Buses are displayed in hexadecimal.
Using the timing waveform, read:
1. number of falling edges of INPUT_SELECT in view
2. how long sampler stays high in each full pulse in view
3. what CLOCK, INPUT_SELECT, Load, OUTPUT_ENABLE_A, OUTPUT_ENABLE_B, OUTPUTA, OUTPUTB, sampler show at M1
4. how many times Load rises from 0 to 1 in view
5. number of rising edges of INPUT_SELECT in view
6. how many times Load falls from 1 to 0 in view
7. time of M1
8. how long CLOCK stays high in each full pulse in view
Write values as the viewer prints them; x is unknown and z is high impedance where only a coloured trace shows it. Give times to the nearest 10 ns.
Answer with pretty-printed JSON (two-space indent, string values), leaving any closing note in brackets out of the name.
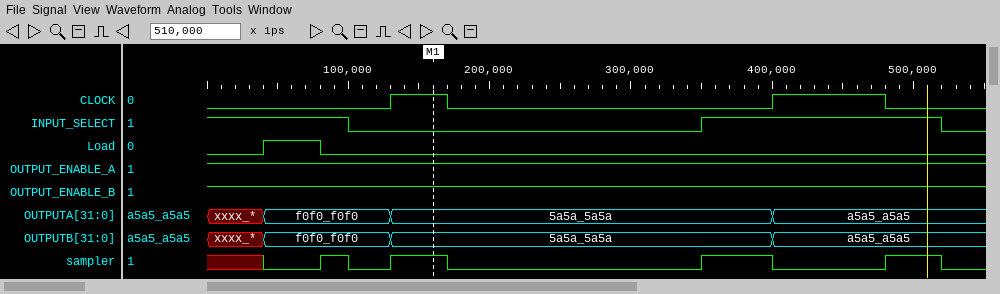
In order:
{
  "number of falling edges of INPUT_SELECT in view": "2",
  "how long sampler stays high in each full pulse in view": "20 ns, 40 ns, 50 ns, 40 ns",
  "what CLOCK, INPUT_SELECT, Load, OUTPUT_ENABLE_A, OUTPUT_ENABLE_B, OUTPUTA, OUTPUTB, sampler show at M1": "CLOCK=1, INPUT_SELECT=0, Load=0, OUTPUT_ENABLE_A=1, OUTPUT_ENABLE_B=1, OUTPUTA=5a5a_5a5a, OUTPUTB=5a5a_5a5a, sampler=1",
  "how many times Load rises from 0 to 1 in view": "1",
  "number of rising edges of INPUT_SELECT in view": "1",
  "how many times Load falls from 1 to 0 in view": "1",
  "time of M1": "160 ns",
  "how long CLOCK stays high in each full pulse in view": "40 ns, 80 ns"
}
